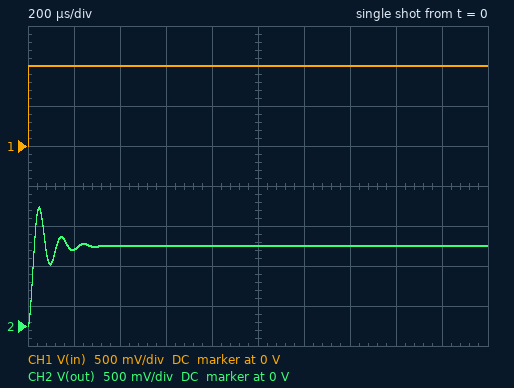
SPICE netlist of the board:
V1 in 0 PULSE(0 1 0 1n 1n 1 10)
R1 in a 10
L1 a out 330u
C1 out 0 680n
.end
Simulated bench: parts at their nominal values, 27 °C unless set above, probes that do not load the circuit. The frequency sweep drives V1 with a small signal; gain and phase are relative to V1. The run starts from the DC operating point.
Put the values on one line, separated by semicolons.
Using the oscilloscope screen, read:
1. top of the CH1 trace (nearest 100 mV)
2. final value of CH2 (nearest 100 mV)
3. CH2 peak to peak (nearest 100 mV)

1.0 V; 1.0 V; 1.5 V
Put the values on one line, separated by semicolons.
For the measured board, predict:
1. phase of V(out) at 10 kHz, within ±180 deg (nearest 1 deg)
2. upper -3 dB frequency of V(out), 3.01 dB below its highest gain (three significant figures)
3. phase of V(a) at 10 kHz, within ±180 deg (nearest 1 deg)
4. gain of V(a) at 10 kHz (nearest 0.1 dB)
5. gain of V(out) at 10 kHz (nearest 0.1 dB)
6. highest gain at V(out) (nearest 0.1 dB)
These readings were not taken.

-75 deg; 12.3 kHz; -75 deg; -11.8 dB; 7.1 dB; 7.1 dB
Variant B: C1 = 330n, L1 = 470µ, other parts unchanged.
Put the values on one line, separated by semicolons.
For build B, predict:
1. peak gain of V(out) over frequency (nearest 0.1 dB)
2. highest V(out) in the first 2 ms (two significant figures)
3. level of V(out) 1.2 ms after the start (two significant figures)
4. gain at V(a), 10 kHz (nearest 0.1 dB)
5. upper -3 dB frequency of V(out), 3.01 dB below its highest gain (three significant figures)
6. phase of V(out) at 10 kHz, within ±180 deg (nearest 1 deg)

11.6 dB; 1.7 V; 1.0 V; -1.1 dB; 14.2 kHz; -28 deg
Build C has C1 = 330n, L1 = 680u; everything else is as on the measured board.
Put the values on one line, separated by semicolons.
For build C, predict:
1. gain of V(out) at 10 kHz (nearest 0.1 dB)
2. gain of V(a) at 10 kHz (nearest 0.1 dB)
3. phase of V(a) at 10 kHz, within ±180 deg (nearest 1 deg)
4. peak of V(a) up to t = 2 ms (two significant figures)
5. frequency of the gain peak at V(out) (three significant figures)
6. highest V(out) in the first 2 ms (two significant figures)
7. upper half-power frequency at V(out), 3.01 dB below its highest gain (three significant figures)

12.5 dB; -6.3 dB; -61 deg; 1.1 V; 10.5 kHz; 1.7 V; 11.6 kHz
